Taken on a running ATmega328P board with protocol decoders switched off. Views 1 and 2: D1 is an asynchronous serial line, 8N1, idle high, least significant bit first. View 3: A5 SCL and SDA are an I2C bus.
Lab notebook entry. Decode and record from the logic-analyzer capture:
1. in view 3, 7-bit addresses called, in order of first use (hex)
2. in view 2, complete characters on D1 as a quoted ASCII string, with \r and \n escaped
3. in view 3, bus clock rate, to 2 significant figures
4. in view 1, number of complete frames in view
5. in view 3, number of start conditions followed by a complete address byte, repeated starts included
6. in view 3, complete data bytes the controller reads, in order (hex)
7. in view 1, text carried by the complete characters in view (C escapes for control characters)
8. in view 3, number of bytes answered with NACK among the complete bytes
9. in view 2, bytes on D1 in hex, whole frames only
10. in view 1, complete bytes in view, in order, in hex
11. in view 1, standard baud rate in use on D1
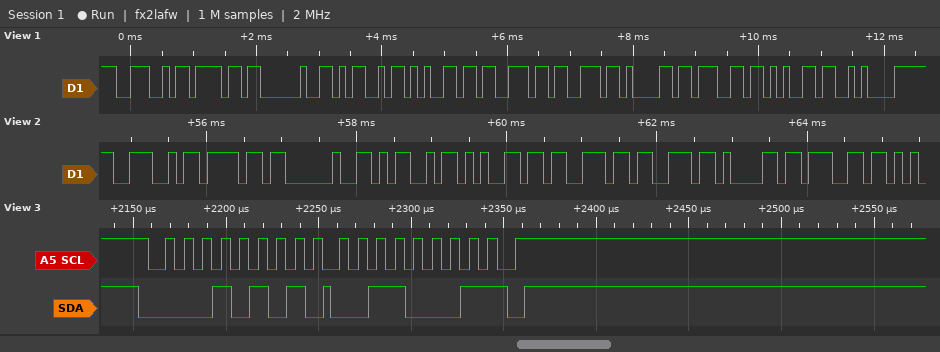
0x0A
"No Messag"
100 kHz
11
1
31
"No Message\n"
1
0x4E 0x6F 0x20 0x4D 0x65 0x73 0x73 0x61 0x67
4E 6F 20 4D 65 73 73 61 67 65 0A
9600 baud
